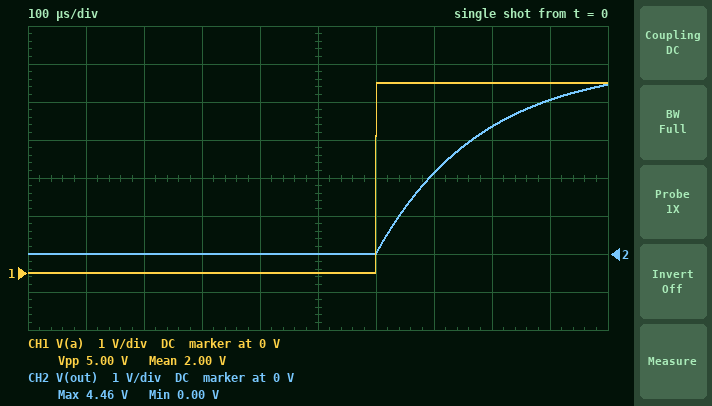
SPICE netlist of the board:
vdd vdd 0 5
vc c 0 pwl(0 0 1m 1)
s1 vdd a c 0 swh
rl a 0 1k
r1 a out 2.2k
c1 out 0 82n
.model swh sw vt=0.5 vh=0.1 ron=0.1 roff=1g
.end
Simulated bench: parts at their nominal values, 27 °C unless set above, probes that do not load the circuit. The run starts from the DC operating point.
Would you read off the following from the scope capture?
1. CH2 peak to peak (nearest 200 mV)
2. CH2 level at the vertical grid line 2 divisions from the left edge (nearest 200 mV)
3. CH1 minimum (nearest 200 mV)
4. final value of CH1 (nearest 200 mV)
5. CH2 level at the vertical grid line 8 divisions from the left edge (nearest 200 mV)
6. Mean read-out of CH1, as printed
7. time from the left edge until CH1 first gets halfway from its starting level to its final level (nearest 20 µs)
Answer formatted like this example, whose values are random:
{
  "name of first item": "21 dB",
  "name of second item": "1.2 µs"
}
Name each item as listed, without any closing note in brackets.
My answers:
{
  "CH2 peak to peak": "4.4 V",
  "CH2 level at the vertical grid line 2 divisions from the left edge": "0 V",
  "CH1 minimum": "0 V",
  "final value of CH1": "5.0 V",
  "CH2 level at the vertical grid line 8 divisions from the left edge": "3.4 V",
  "Mean read-out of CH1, as printed": "2.00 V",
  "time from the left edge until CH1 first gets halfway from its starting level to its final level": "600 µs"
}
